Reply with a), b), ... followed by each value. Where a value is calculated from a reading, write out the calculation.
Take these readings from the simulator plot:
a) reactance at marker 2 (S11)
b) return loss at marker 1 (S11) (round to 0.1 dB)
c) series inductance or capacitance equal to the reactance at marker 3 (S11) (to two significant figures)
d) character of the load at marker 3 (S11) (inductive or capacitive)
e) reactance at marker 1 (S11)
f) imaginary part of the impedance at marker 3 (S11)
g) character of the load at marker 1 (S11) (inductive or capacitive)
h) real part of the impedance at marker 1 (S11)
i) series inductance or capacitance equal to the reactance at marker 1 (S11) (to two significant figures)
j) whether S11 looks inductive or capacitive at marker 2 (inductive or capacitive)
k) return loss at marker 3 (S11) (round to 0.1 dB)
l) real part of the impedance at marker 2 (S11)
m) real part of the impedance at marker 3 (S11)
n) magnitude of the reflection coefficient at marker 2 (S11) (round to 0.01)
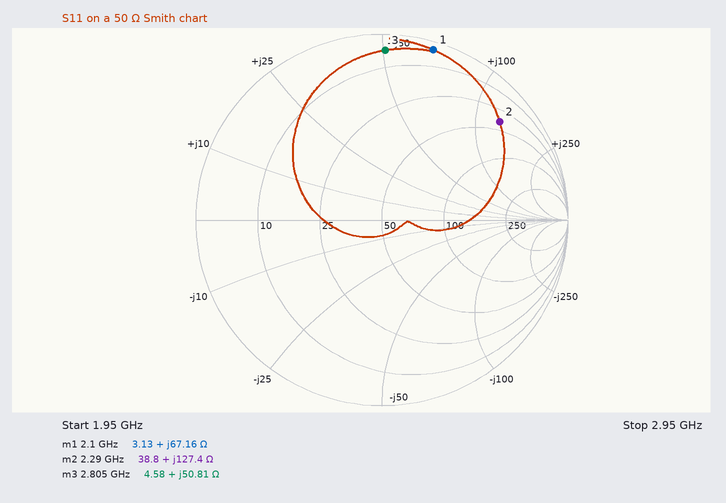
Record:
a) +127.4 Ω
b) 0.4 dB
c) L = 50.81 Ω/(2π × 2.805 GHz) ≈ 2.9 nH
d) inductive
e) +67.16 Ω
f) +50.81 Ω
g) inductive
h) 3.13 Ω
i) L = 67.16 Ω/(2π × 2.1 GHz) ≈ 5.1 nH
j) inductive
k) 0.8 dB
l) 38.8 Ω
m) 4.58 Ω
n) 0.82
